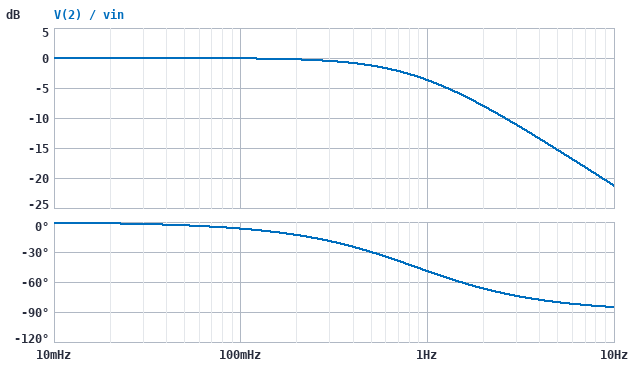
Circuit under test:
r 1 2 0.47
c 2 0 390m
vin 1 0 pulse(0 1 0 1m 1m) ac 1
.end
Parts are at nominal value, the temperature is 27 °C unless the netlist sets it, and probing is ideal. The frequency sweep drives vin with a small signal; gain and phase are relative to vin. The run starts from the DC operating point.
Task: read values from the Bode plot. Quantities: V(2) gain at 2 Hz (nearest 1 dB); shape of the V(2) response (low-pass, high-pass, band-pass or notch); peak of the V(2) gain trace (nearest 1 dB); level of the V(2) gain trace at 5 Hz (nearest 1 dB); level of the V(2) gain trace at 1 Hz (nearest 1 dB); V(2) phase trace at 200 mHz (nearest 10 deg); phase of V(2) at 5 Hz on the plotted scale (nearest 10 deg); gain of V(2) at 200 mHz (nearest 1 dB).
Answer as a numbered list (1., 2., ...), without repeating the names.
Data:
1. -8 dB
2. low-pass
3. 0 dB
4. -15 dB
5. -4 dB
6. -10 deg
7. -80 deg
8. 0 dB
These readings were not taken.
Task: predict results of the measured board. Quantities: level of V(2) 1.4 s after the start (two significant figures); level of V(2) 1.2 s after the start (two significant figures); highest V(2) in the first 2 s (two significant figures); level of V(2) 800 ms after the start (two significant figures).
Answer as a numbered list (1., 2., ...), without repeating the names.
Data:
1. 1.0 V
2. 1.0 V
3. 1.0 V
4. 990 mV
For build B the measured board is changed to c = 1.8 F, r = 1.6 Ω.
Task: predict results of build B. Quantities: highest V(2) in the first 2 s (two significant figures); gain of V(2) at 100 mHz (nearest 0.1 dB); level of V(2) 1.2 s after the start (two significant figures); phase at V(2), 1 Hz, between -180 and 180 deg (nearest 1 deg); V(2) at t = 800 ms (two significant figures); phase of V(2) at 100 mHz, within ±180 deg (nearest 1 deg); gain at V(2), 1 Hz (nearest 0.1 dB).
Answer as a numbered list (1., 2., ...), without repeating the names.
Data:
1. 500 mV
2. -6.3 dB
3. 340 mV
4. -87 deg
5. 240 mV
6. -61 deg
7. -25.2 dB
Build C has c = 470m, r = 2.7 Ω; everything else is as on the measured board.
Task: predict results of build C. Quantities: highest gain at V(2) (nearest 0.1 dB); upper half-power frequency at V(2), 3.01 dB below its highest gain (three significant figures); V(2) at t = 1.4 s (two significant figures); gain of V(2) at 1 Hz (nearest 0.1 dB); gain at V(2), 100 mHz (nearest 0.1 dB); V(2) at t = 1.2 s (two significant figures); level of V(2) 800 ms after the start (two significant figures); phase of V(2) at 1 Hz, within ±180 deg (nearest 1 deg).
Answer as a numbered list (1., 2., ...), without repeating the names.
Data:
1. 0 dB
2. 125 mHz
3. 670 mV
4. -18.1 dB
5. -2.1 dB
6. 610 mV
7. 470 mV
8. -83 deg
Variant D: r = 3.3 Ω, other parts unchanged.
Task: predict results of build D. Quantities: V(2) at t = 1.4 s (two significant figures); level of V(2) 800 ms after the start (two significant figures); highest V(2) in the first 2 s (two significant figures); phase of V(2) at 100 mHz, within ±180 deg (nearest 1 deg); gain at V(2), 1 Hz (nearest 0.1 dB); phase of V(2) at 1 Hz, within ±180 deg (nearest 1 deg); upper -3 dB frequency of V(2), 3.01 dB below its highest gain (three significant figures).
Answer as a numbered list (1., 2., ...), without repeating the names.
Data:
1. 660 mV
2. 460 mV
3. 790 mV
4. -39 deg
5. -18.2 dB
6. -83 deg
7. 124 mHz
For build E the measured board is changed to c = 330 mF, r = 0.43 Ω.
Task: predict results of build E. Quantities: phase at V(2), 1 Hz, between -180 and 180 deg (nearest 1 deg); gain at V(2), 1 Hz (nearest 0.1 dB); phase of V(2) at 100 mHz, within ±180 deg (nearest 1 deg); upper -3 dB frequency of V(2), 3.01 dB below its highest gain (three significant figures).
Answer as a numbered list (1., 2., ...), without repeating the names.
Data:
1. -42 deg
2. -2.5 dB
3. -5 deg
4. 1.12 Hz
